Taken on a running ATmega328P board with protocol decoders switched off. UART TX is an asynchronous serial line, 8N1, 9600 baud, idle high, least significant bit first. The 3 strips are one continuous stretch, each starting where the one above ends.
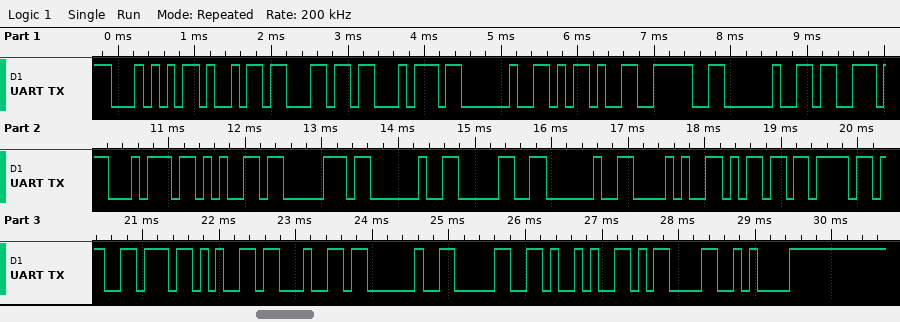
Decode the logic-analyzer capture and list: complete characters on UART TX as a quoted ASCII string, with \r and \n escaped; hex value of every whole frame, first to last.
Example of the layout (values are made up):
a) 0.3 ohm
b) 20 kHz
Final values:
a) "Tilt -> step 0 (moved 0)\r\n"
b) 54 69 6C 74 20 2D 3E 20 73 74 65 70 20 30 20 28 6D 6F 76 65 64 20 30 29 0D 0A
